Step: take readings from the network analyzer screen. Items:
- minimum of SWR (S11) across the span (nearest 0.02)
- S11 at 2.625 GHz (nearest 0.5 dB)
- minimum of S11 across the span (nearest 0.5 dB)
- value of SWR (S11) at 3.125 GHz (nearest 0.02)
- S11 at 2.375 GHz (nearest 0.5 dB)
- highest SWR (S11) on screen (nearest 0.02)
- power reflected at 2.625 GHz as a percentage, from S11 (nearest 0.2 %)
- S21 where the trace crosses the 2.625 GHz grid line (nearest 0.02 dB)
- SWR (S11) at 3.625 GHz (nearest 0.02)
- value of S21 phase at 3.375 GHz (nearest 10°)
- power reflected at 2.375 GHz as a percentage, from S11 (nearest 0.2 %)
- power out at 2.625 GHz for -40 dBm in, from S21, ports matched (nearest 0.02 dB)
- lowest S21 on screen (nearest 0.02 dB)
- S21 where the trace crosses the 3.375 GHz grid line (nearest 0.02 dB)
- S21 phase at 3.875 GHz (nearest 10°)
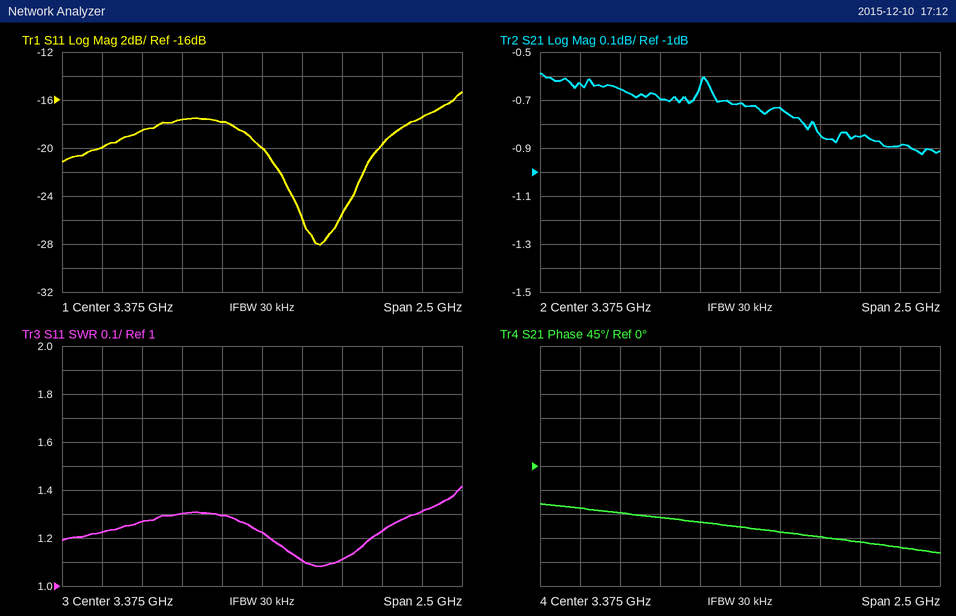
1.08
-18.5 dB
-28.0 dB
1.30
-20.0 dB
1.42
1.4 %
-0.66 dB
1.10
-110°
1.0 %
-40.66 dBm
-0.92 dB
-0.72 dB
-130°
